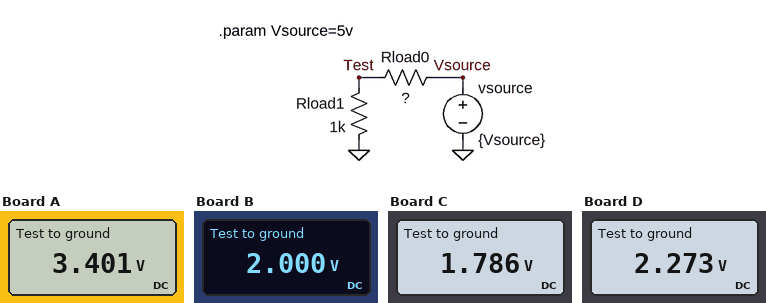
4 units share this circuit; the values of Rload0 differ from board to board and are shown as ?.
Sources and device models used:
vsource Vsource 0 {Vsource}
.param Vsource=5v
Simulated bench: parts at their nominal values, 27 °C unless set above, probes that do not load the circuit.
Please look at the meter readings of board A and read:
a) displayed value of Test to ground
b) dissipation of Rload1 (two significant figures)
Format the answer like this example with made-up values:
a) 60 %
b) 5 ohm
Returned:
a) 3.401 V
b) 12 mW
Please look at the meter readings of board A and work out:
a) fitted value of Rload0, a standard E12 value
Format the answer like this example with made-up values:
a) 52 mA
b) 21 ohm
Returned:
a) 470 Ω
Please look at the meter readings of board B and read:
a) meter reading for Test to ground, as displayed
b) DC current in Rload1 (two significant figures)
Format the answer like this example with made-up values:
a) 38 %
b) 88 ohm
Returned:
a) 2.000 V
b) 2.0 mA
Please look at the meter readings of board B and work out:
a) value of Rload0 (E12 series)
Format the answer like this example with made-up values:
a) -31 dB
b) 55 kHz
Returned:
a) 1.5 kΩ
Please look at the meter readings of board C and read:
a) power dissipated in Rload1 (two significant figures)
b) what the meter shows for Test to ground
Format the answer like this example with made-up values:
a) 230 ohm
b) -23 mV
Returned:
a) 3.2 mW
b) 1.786 V
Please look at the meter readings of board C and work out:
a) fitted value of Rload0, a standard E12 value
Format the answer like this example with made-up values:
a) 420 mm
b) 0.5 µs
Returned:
a) 1.8 kΩ
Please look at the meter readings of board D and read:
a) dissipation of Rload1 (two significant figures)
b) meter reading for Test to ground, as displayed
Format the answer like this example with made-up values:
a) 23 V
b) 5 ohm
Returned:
a) 5.2 mW
b) 2.273 V
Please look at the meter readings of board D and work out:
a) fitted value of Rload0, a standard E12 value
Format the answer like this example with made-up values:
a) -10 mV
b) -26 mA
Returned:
a) 1.2 kΩ
